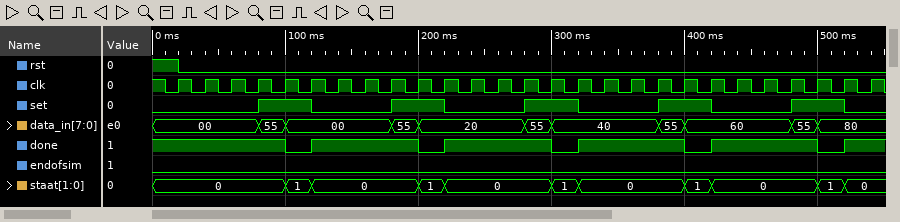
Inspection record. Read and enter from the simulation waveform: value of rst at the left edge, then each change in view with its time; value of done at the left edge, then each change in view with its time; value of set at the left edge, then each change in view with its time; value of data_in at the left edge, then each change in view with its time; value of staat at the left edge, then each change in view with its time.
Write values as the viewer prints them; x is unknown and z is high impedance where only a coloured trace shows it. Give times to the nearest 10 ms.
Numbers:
1, 0 at 20 ms
1, 0 at 100 ms, 1 at 120 ms, 0 at 200 ms, 1 at 220 ms, 0 at 300 ms, 1 at 320 ms, 0 at 400 ms, 1 at 420 ms, 0 at 500 ms, 1 at 520 ms
0, 1 at 80 ms, 0 at 120 ms, 1 at 180 ms, 0 at 220 ms, 1 at 280 ms, 0 at 320 ms, 1 at 380 ms, 0 at 420 ms, 1 at 480 ms, 0 at 520 ms
00, 55 at 80 ms, 00 at 100 ms, 55 at 180 ms, 20 at 200 ms, 55 at 280 ms, 40 at 300 ms, 55 at 380 ms, 60 at 400 ms, 55 at 480 ms, 80 at 500 ms
0, 1 at 100 ms, 0 at 120 ms, 1 at 200 ms, 0 at 220 ms, 1 at 300 ms, 0 at 320 ms, 1 at 400 ms, 0 at 420 ms, 1 at 500 ms, 0 at 520 ms
